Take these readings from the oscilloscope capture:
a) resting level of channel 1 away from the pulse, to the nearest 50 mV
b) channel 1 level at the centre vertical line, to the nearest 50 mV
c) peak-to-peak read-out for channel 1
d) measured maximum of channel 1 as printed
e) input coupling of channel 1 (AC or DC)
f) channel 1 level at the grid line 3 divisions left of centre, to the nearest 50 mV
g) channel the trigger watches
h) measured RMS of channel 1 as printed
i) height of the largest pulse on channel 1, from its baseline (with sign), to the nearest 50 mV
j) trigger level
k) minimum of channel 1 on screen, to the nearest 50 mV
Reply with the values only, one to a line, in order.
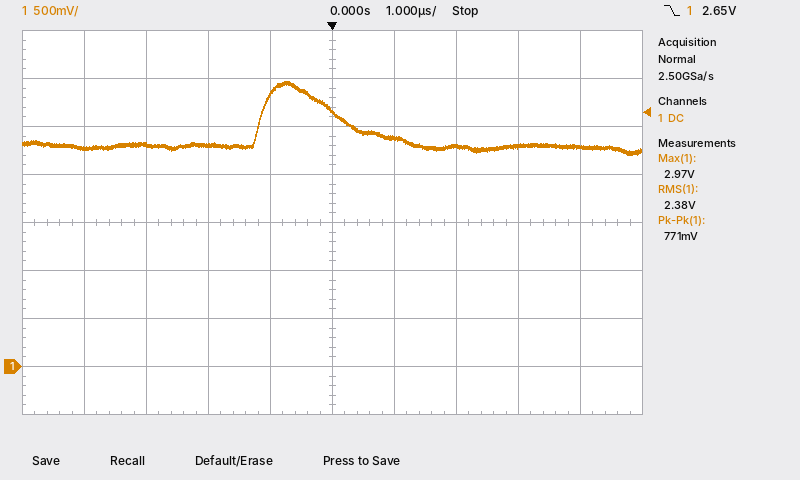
2.30 V
2.65 V
771 mV
2.97 V
DC
2.30 V
channel 1
2.38 V
+700 mV
2.65 V
2.20 V
